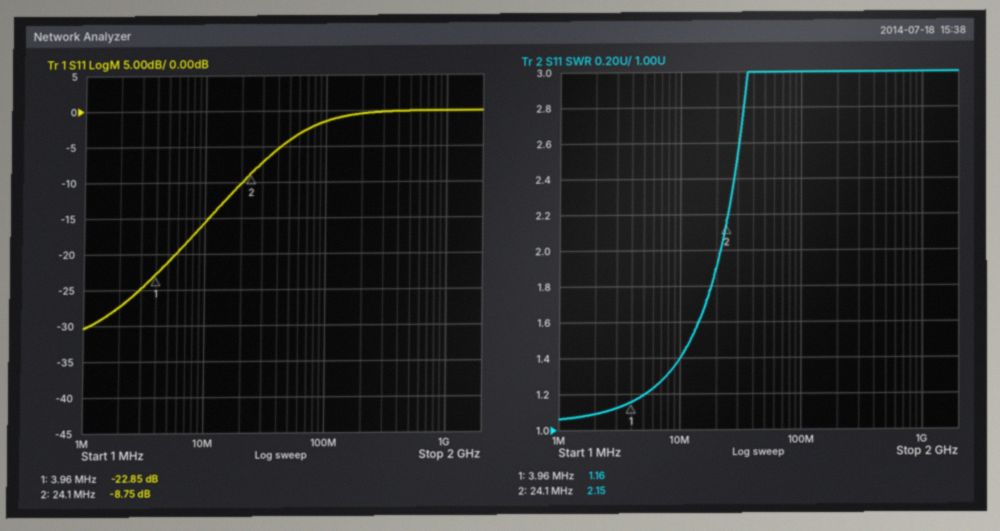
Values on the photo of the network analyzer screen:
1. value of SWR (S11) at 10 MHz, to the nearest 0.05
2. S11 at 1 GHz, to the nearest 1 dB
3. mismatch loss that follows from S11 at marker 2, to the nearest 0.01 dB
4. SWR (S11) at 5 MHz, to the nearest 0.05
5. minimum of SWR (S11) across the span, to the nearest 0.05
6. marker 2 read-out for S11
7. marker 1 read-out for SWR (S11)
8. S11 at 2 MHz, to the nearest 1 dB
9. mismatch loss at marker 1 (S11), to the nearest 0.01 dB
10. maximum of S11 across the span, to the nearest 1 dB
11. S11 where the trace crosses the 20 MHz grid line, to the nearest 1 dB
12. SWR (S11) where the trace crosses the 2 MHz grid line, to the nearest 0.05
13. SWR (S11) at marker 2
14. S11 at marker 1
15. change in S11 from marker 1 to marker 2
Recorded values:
1.40
0 dB
0.62 dB
1.20
1.05
-8.75 dB
1.16
-27 dB
0.02 dB
0 dB
-10 dB
1.10
2.15
-22.85 dB
14.10 dB
